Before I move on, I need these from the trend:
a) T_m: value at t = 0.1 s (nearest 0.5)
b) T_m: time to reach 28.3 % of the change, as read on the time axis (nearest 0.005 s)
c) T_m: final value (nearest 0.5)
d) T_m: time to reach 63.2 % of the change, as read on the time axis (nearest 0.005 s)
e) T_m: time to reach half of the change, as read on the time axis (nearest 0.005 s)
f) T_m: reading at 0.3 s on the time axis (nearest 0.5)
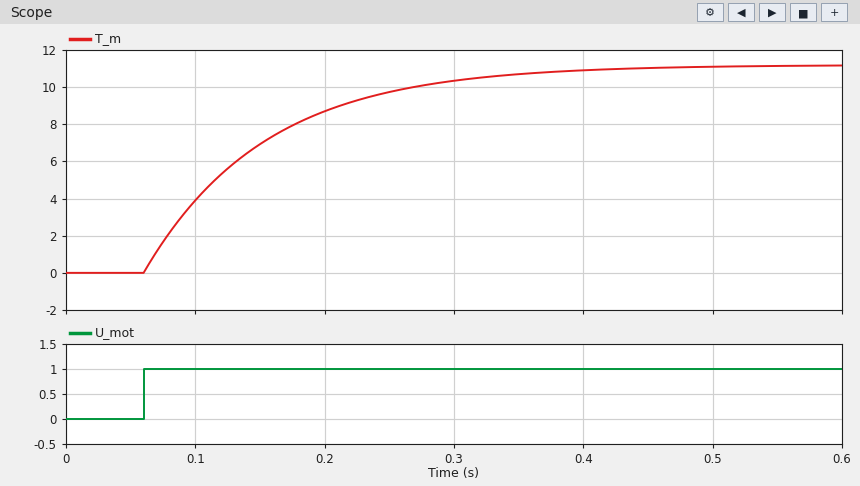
4.0
0.090 s
11.0
0.155 s
0.125 s
10.5
